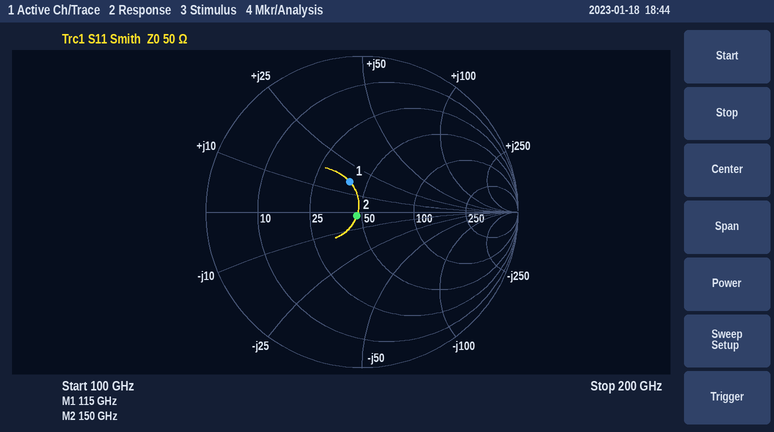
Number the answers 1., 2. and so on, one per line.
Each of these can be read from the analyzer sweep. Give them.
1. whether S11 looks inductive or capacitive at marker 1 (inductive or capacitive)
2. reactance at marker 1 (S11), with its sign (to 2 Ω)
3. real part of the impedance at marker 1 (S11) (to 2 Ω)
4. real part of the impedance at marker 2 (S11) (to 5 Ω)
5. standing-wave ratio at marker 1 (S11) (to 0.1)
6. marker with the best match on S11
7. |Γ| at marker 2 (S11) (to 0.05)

1. inductive
2. +16 Ω
3. 40 Ω
4. 45 Ω
5. 1.5
6. marker 2
7. 0.05
